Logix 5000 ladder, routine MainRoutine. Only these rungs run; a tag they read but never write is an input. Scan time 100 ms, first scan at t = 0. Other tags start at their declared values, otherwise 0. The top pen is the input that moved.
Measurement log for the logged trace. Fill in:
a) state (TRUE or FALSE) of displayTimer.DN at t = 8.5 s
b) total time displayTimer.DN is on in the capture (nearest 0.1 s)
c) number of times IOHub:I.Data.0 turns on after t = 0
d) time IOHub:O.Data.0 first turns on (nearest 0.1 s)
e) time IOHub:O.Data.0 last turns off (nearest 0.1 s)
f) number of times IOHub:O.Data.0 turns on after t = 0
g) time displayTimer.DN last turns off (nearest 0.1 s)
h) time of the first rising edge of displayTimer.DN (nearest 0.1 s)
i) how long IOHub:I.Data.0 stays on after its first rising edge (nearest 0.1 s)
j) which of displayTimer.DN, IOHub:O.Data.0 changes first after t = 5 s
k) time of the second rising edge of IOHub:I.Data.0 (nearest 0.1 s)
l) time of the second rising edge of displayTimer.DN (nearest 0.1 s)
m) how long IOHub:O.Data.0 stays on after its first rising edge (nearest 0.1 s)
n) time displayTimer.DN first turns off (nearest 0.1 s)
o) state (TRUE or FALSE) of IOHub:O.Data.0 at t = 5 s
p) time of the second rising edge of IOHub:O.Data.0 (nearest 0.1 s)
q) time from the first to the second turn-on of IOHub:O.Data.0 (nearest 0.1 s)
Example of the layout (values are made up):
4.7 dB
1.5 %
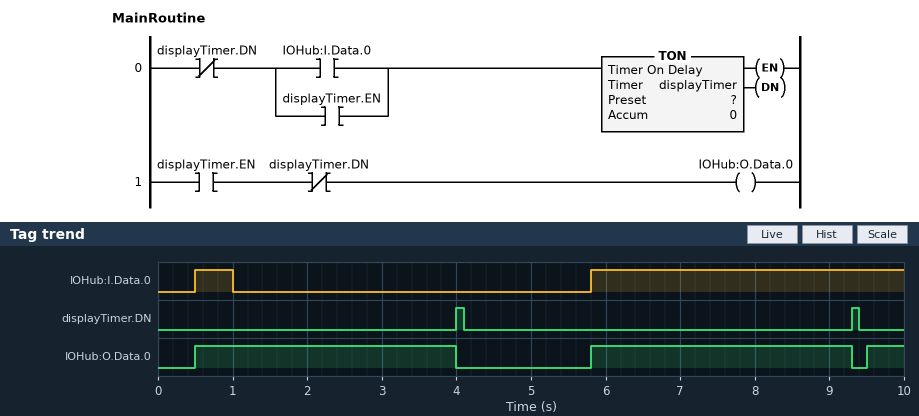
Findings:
FALSE
0.2 s
2
0.5 s
9.3 s
3
9.4 s
4.0 s
0.5 s
IOHub:O.Data.0
5.8 s
9.3 s
3.5 s
4.1 s
FALSE
5.8 s
5.3 s
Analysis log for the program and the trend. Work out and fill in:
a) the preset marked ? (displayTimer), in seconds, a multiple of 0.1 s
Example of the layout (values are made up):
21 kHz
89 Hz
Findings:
3.5 s
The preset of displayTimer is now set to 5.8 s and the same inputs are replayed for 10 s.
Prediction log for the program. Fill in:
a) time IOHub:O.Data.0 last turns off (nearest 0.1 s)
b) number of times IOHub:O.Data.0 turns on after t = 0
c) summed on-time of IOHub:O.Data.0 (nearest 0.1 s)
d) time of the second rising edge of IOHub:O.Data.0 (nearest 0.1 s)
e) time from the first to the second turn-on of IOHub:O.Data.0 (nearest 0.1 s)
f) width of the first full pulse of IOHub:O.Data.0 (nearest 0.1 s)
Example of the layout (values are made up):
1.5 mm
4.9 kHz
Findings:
6.3 s
2
9.3 s
6.5 s
6.0 s
5.8 s
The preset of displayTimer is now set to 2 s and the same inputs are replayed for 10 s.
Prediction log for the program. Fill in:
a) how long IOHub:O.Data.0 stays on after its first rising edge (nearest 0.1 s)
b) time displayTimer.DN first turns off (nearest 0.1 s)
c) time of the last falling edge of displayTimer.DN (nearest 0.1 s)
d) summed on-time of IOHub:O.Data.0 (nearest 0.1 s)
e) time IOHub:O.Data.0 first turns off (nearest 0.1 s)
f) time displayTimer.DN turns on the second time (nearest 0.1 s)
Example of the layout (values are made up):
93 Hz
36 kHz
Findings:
2.0 s
2.6 s
7.9 s
6.0 s
2.5 s
7.8 s
